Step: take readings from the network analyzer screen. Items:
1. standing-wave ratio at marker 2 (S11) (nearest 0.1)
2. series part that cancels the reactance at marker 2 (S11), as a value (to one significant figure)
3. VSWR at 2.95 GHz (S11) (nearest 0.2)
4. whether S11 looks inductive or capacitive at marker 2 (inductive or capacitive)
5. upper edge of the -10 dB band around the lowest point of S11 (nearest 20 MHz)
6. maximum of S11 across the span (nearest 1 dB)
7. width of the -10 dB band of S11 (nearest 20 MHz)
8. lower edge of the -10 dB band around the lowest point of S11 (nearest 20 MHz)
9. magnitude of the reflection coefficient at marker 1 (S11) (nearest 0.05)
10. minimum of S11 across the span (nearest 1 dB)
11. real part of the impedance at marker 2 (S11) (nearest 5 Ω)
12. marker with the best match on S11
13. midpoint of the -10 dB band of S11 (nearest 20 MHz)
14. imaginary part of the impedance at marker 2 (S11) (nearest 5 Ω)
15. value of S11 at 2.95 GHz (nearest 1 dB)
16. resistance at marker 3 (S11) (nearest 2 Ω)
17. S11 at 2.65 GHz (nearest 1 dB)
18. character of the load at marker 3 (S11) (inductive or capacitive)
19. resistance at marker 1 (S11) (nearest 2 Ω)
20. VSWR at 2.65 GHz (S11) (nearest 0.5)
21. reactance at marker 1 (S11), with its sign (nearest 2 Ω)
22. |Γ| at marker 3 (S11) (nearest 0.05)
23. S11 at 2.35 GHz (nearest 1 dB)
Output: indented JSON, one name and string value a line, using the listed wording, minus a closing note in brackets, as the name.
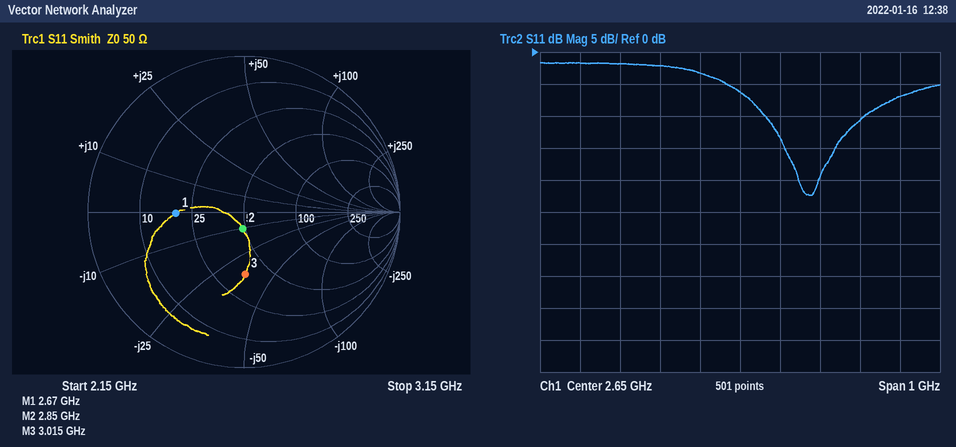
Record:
{
  "standing-wave ratio at marker 2 (S11)": "1.2",
  "series part that cancels the reactance at marker 2 (S11), as a value": "600 pH",
  "VSWR at 2.95 GHz (S11)": "1.8",
  "whether S11 looks inductive or capacitive at marker 2": "capacitive",
  "upper edge of the -10 dB band around the lowest point of S11": "2.96 GHz",
  "maximum of S11 across the span": "-2 dB",
  "width of the -10 dB band of S11": "240 MHz",
  "lower edge of the -10 dB band around the lowest point of S11": "2.72 GHz",
  "magnitude of the reflection coefficient at marker 1 (S11)": "0.45",
  "minimum of S11 across the span": "-22 dB",
  "real part of the impedance at marker 2 (S11)": "50 Ω",
  "marker with the best match on S11": "marker 2",
  "midpoint of the -10 dB band of S11": "2.84 GHz",
  "imaginary part of the impedance at marker 2 (S11)": "-10 Ω",
  "value of S11 at 2.95 GHz": "-11 dB",
  "resistance at marker 3 (S11)": "36 Ω",
  "S11 at 2.65 GHz": "-6 dB",
  "character of the load at marker 3 (S11)": "capacitive",
  "resistance at marker 1 (S11)": "20 Ω",
  "VSWR at 2.65 GHz (S11)": "3.0",
  "reactance at marker 1 (S11), with its sign": "0 Ω",
  "|Γ| at marker 3 (S11)": "0.40",
  "S11 at 2.35 GHz": "-2 dB"
}
